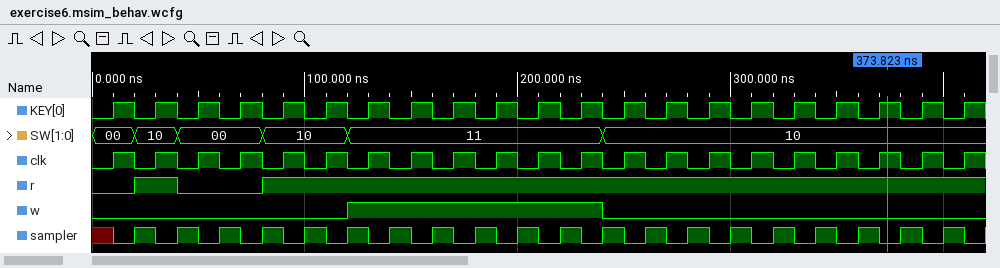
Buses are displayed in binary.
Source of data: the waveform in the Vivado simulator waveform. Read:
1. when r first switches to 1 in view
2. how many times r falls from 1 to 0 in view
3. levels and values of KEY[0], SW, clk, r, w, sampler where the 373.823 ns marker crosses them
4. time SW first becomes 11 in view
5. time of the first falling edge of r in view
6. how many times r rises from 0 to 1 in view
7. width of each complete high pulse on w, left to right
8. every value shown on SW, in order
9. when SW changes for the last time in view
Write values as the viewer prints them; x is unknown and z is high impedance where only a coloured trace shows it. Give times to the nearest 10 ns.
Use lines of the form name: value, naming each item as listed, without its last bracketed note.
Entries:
when r first switches to 1 in view: 20 ns
how many times r falls from 1 to 0 in view: 1
levels and values of KEY[0], SW, clk, r, w, sampler where the 373.823 ns marker crosses them: KEY[0]=1, SW=10, clk=1, r=1, w=0, sampler=0
time SW first becomes 11 in view: 120 ns
time of the first falling edge of r in view: 40 ns
how many times r rises from 0 to 1 in view: 2
width of each complete high pulse on w, left to right: 120 ns
every value shown on SW, in order: 00, 10, 00, 10, 11, 10
when SW changes for the last time in view: 240 ns
